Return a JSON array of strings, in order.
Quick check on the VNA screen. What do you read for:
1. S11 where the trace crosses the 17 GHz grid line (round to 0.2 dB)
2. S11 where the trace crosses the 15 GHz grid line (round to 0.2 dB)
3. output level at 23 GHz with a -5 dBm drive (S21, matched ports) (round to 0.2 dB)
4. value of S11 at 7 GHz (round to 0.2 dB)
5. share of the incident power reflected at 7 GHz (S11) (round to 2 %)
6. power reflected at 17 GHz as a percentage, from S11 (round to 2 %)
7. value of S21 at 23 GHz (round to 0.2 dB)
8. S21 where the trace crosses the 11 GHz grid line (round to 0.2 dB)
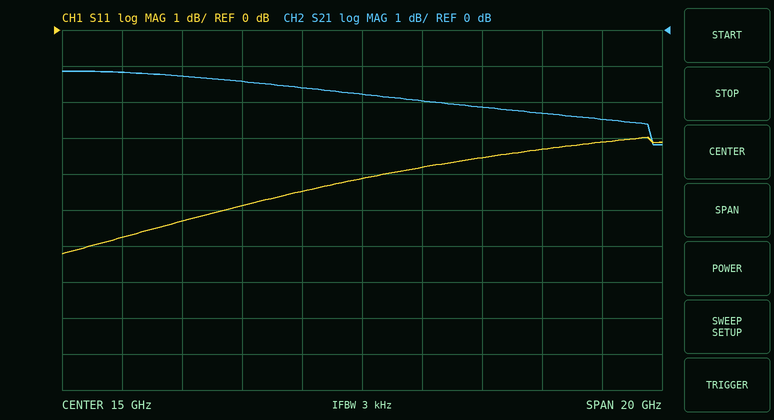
["-3.8 dB", "-4.2 dB", "-7.4 dBm", "-5.8 dB", "26 %", "42 %", "-2.4 dB", "-1.4 dB"]
